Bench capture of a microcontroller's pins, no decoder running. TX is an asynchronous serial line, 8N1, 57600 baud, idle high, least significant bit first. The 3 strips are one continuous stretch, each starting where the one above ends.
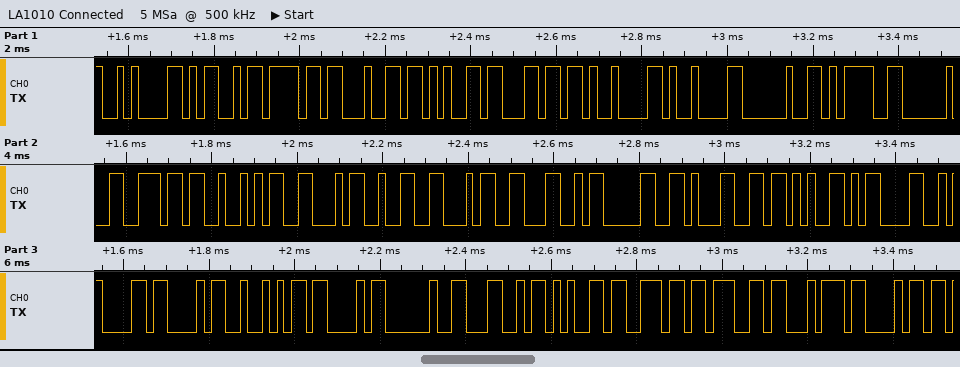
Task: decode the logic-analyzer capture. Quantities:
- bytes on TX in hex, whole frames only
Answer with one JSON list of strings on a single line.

["0A 4D 6F 64 65 6C 09 09 20 3D 20 6E 52 46 32 34 4C 30 31 2B 0D 0A 43 52 43 20 4C 65 6E 67 74 68"]
